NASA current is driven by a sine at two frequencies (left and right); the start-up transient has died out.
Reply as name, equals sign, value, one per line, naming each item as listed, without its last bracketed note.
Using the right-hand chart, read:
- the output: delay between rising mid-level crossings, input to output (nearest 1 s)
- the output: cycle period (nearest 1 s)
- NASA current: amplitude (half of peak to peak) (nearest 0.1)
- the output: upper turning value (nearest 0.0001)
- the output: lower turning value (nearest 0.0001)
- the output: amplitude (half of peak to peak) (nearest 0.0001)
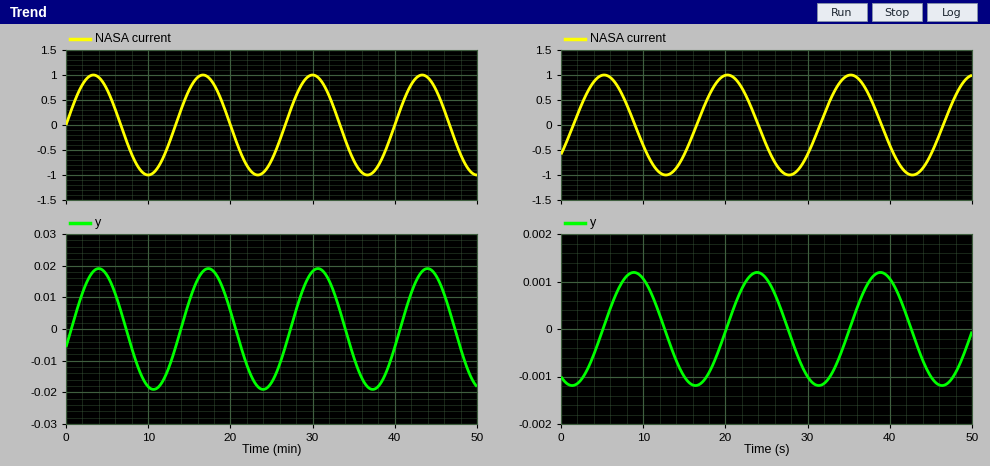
the output: delay between rising mid-level crossings, input to output = 4 s
the output: cycle period = 15 s
NASA current: amplitude (half of peak to peak) = 1.0
the output: upper turning value = 0.0012
the output: lower turning value = -0.0012
the output: amplitude (half of peak to peak) = 0.0012
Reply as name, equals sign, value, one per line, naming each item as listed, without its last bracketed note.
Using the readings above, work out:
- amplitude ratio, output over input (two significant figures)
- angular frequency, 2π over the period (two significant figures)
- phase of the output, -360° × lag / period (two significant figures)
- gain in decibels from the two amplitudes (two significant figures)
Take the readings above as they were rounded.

amplitude ratio, output over input = 0.0012
angular frequency, 2π over the period = 0.42 rad/s
phase of the output, -360° × lag / period = -96°
gain in decibels from the two amplitudes = -58 dB
